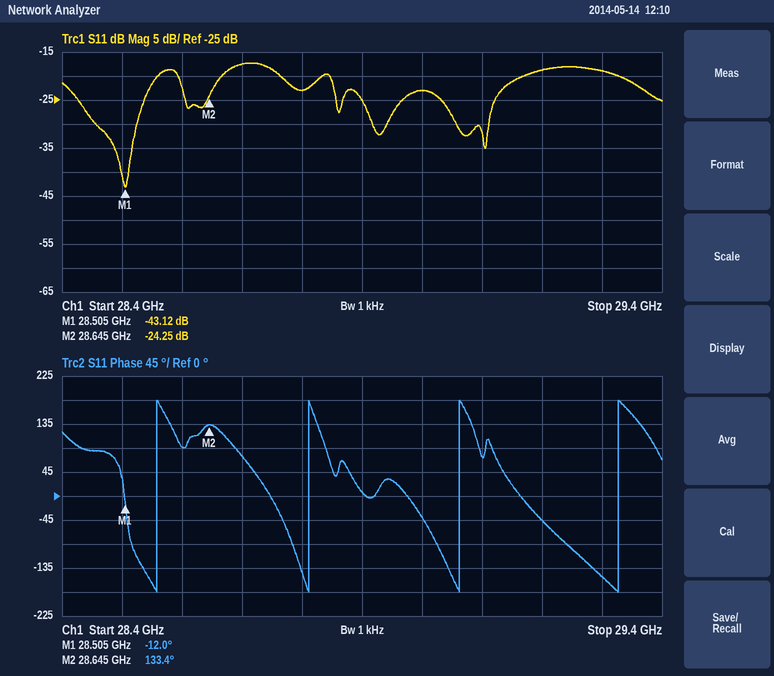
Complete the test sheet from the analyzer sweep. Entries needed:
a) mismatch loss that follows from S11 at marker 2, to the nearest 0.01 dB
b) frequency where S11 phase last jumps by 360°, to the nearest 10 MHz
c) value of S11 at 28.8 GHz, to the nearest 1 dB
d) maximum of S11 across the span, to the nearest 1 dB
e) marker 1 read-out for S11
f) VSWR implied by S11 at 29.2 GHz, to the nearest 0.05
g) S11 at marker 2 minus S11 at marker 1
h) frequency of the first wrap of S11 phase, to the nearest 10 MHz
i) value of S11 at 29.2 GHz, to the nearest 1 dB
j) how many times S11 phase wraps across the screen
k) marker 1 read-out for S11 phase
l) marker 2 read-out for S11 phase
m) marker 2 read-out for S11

0.02 dB
29.33 GHz
-23 dB
-17 dB
-43.12 dB
1.25
18.87 dB
28.56 GHz
-19 dB
4
-12.0°
133.4°
-24.25 dB
